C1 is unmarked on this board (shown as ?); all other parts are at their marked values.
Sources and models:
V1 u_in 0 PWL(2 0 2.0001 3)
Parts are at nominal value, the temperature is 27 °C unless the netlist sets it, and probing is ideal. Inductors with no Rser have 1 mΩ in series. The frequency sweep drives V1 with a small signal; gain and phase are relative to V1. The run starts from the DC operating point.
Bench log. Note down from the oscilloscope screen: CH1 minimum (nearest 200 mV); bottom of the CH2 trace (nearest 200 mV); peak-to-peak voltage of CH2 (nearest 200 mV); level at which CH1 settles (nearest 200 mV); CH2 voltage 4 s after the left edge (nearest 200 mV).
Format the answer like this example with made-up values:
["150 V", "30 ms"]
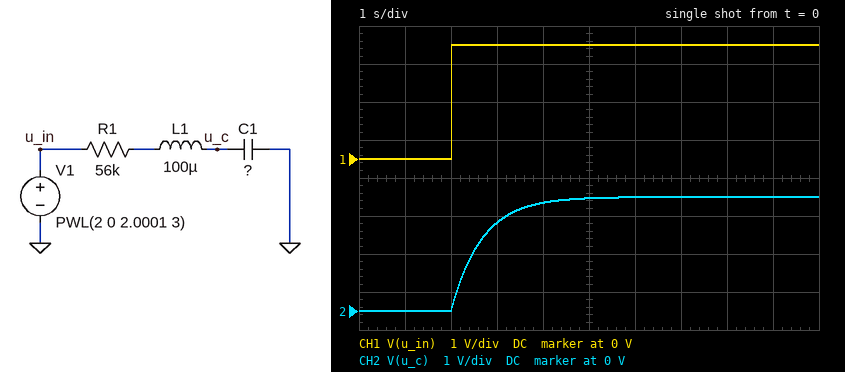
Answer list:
["0 V", "0 V", "3.0 V", "3.0 V", "2.8 V"]
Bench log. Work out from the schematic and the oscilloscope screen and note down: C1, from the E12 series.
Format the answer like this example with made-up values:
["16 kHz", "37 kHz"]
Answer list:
["12 µF"]
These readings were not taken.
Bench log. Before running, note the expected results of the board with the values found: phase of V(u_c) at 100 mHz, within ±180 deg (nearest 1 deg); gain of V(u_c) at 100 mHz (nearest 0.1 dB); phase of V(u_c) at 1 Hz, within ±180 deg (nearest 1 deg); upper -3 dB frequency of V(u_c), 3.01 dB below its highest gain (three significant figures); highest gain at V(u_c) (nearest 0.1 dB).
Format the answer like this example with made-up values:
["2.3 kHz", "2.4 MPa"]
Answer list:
["-23 deg", "-0.7 dB", "-77 deg", "237 mHz", "0 dB"]
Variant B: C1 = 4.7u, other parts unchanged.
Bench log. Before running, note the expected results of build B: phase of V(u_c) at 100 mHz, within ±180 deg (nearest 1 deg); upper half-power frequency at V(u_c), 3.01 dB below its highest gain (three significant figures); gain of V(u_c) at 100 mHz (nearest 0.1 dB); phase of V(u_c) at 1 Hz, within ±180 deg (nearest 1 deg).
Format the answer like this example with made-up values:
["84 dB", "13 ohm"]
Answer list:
["-9 deg", "605 mHz", "-0.1 dB", "-59 deg"]
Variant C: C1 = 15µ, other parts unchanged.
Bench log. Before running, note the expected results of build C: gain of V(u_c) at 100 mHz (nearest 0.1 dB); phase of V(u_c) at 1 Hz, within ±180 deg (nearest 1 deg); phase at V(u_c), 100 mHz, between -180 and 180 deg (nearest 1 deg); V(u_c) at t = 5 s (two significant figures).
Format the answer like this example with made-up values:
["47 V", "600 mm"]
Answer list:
["-1.1 dB", "-79 deg", "-28 deg", "2.9 V"]
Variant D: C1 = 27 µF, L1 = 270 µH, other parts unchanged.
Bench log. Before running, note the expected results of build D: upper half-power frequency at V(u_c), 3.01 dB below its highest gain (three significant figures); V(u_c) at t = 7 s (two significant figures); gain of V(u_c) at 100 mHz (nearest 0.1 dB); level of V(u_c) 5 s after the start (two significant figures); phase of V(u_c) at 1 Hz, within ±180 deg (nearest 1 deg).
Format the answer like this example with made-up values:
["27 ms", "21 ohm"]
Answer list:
["105 mHz", "2.9 V", "-2.8 dB", "2.6 V", "-84 deg"]
